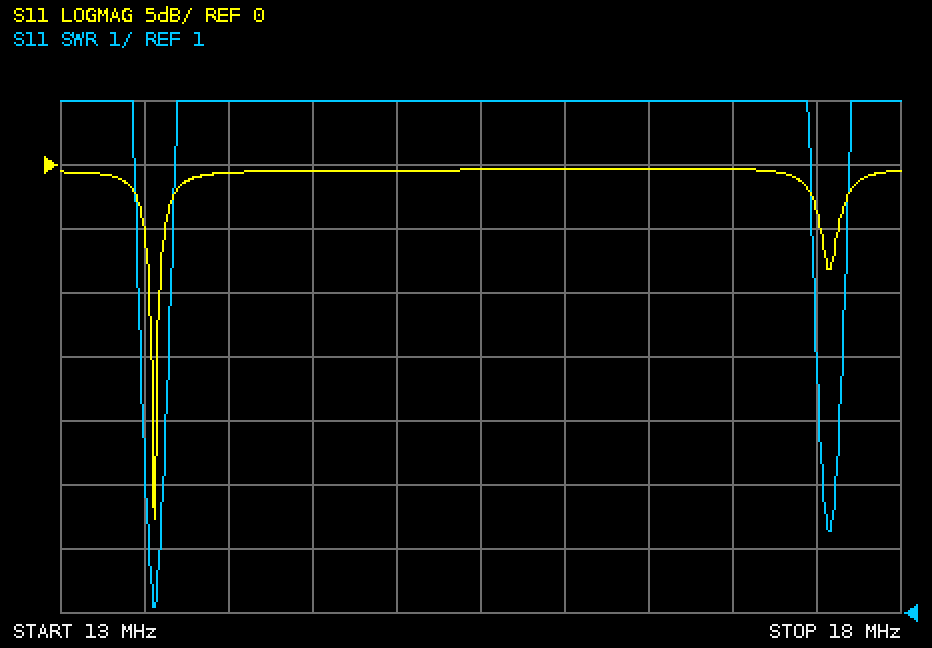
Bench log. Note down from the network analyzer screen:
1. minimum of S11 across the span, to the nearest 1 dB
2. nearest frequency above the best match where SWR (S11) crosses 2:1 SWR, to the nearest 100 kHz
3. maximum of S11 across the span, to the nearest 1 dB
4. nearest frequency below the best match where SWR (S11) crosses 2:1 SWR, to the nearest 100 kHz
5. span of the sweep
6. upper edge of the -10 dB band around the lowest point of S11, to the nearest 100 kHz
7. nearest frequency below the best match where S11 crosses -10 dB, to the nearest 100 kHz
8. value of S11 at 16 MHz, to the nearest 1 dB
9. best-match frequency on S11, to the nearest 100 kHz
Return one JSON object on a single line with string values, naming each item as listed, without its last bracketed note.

{"minimum of S11 across the span, to the nearest 1 dB": "-28 dB", "nearest frequency above the best match where SWR (S11) crosses 2:1 SWR, to the nearest 100 kHz": "13.6 MHz", "maximum of S11 across the span, to the nearest 1 dB": "0 dB", "nearest frequency below the best match where SWR (S11) crosses 2:1 SWR, to the nearest 100 kHz": "13.5 MHz", "span of the sweep": "5 MHz", "upper edge of the -10 dB band around the lowest point of S11, to the nearest 100 kHz": "13.6 MHz", "nearest frequency below the best match where S11 crosses -10 dB, to the nearest 100 kHz": "13.5 MHz", "value of S11 at 16 MHz, to the nearest 1 dB": "0 dB", "best-match frequency on S11, to the nearest 100 kHz": "13.6 MHz"}
